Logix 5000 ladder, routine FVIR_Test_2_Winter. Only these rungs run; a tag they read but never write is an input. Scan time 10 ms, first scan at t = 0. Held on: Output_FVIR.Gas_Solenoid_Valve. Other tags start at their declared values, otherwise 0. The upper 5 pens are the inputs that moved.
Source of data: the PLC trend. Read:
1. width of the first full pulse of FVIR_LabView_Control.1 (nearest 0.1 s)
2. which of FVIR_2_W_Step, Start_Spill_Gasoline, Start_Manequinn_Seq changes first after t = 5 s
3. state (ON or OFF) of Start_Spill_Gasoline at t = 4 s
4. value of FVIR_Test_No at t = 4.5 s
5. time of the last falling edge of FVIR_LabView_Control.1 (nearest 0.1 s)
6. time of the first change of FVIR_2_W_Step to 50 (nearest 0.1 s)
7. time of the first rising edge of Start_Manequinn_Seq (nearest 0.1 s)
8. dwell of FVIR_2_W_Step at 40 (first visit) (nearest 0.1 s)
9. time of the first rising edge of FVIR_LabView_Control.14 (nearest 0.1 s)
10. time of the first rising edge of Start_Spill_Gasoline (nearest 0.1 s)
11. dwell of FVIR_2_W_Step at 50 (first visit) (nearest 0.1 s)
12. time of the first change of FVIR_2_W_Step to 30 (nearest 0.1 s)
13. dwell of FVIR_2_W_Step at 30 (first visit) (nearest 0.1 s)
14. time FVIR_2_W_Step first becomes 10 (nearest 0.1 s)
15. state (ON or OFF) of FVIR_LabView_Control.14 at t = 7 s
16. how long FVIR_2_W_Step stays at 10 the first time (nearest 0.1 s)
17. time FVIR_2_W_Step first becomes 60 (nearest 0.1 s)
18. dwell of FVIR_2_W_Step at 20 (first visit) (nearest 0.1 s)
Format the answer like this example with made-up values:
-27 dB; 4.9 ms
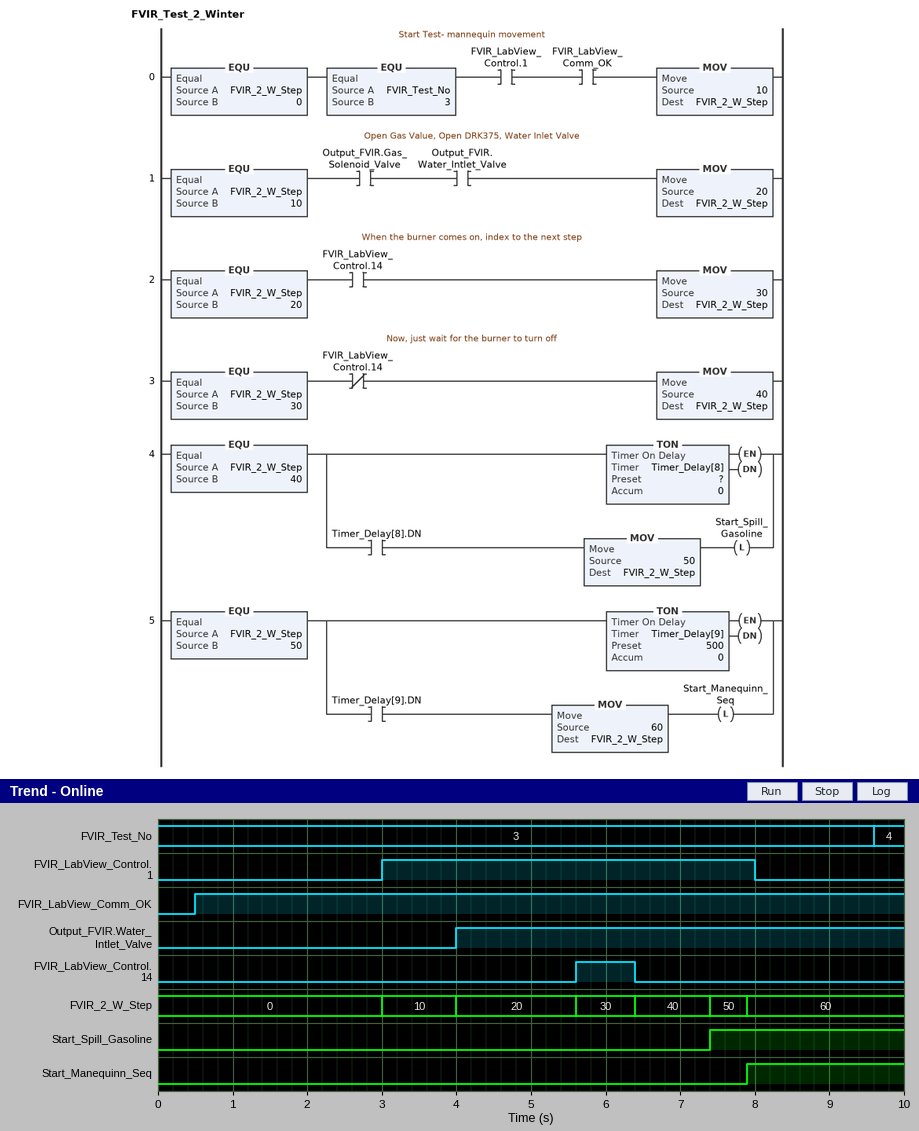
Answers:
5.0 s; FVIR_2_W_Step; OFF; 3; 8.0 s; 7.4 s; 7.9 s; 1.0 s; 5.6 s; 7.4 s; 0.5 s; 5.6 s; 0.8 s; 3.0 s; OFF; 1.0 s; 7.9 s; 1.6 s
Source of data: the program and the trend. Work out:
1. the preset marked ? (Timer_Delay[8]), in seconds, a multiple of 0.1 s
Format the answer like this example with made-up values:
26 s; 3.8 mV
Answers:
1.0 s
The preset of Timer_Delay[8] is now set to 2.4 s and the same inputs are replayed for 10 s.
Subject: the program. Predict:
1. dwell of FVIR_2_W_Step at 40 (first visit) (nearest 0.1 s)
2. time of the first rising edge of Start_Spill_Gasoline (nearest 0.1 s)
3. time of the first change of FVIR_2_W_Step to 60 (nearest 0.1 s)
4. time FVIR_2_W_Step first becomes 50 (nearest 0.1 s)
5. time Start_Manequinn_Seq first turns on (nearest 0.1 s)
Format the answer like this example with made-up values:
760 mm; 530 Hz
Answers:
2.4 s; 8.8 s; 9.3 s; 8.8 s; 9.3 s
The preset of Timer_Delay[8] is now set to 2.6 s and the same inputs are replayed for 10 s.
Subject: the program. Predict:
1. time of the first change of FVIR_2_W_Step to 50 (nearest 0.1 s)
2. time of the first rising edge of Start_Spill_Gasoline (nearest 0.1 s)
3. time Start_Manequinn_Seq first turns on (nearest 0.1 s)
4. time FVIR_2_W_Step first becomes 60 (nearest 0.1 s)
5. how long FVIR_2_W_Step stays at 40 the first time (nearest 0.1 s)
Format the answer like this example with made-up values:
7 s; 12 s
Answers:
9.0 s; 9.0 s; 9.5 s; 9.5 s; 2.6 s
